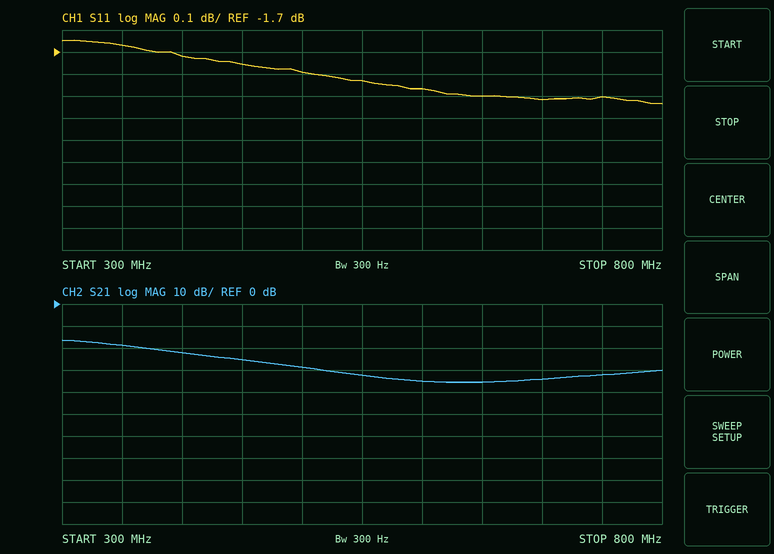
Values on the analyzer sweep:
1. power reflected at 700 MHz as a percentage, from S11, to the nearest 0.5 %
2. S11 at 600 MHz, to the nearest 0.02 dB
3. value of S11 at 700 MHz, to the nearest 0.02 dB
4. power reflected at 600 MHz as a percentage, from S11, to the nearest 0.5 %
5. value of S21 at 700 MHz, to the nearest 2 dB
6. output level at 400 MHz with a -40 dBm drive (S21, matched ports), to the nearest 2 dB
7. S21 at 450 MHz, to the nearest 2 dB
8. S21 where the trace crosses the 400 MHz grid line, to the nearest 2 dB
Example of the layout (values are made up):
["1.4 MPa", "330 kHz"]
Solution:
["64.5 %", "-1.86 dB", "-1.92 dB", "65.0 %", "-34 dB", "-62 dBm", "-26 dB", "-22 dB"]
